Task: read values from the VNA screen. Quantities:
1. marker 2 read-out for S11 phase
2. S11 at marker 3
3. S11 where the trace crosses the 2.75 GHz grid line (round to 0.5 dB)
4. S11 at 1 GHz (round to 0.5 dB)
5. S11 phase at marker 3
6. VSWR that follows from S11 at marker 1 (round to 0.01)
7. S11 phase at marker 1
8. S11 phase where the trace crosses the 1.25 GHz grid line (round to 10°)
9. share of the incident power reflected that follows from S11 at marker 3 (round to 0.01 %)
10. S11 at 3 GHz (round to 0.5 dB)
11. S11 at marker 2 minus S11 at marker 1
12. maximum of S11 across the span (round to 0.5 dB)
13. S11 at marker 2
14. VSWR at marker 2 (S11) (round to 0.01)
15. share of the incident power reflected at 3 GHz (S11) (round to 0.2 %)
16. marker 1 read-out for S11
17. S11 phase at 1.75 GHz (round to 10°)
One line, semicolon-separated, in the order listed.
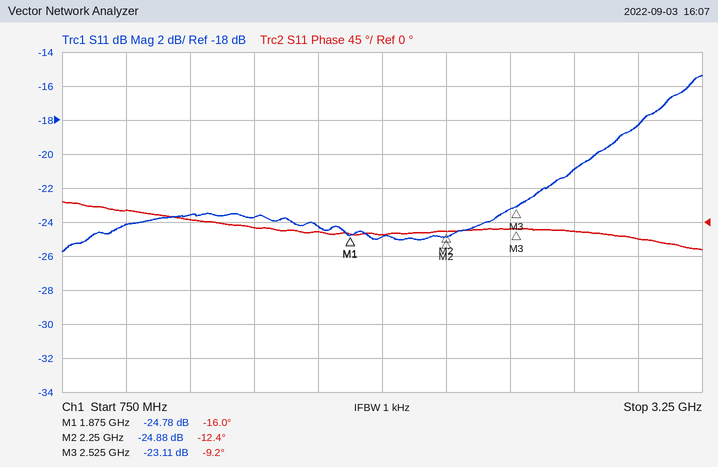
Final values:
-12.4°; -23.11 dB; -21.0 dB; -24.0 dB; -9.2°; 1.12; -16.0°; 0°; 0.49 %; -18.5 dB; -0.10 dB; -15.5 dB; -24.88 dB; 1.12; 1.4 %; -24.78 dB; -10°
